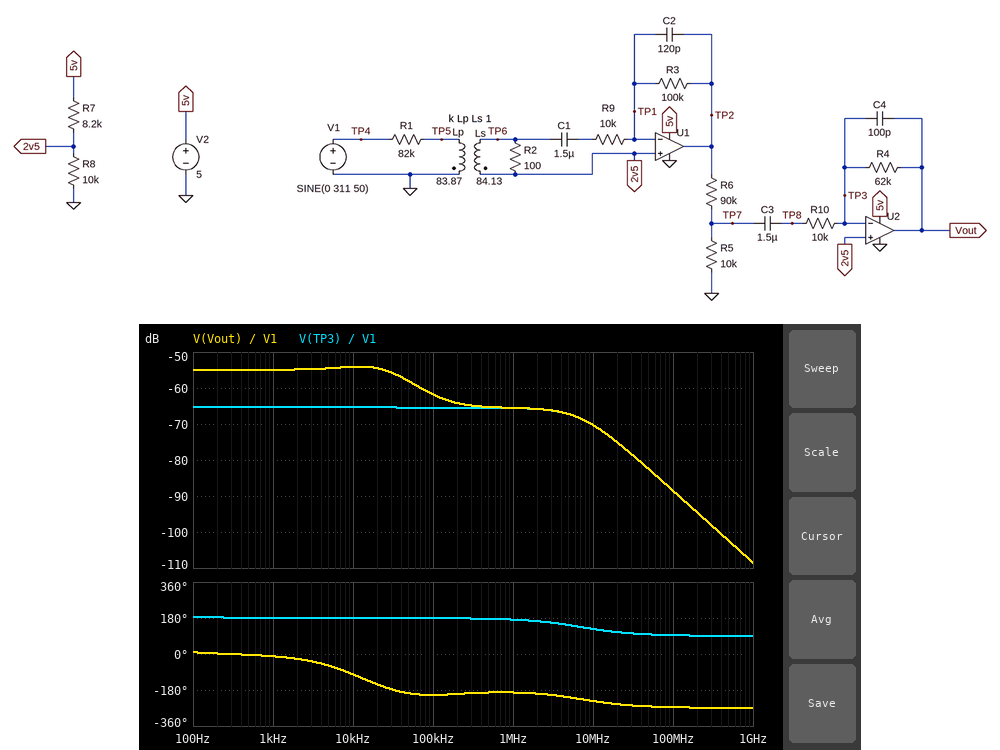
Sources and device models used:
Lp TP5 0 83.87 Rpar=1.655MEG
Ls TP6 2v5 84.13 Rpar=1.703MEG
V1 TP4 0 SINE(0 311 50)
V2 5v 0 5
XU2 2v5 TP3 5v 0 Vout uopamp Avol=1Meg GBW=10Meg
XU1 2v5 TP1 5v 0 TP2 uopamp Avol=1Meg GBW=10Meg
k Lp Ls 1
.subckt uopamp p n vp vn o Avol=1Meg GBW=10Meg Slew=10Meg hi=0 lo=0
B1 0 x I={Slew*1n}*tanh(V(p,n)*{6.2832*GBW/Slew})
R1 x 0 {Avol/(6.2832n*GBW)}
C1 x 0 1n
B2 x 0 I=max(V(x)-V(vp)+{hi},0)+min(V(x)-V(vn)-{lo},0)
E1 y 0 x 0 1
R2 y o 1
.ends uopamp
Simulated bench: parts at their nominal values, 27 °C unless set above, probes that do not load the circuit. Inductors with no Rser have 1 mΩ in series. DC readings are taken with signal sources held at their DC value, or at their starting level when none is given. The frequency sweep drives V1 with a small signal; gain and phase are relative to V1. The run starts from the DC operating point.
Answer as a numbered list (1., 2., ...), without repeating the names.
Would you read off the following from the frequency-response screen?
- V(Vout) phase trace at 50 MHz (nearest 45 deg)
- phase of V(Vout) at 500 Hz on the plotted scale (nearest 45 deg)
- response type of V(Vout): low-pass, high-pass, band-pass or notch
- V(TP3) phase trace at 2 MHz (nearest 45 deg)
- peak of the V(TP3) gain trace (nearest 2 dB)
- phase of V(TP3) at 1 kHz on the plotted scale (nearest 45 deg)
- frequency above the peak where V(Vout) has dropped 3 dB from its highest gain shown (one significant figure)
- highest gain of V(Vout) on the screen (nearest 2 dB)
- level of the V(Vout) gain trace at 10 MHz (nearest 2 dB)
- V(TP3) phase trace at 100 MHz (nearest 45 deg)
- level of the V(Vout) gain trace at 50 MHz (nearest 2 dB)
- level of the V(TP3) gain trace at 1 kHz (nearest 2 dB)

1. -270 deg
2. 0 deg
3. low-pass
4. 180 deg
5. -66 dB
6. 180 deg
7. 40 kHz
8. -54 dB
9. -70 dB
10. 90 deg
11. -82 dB
12. -66 dB
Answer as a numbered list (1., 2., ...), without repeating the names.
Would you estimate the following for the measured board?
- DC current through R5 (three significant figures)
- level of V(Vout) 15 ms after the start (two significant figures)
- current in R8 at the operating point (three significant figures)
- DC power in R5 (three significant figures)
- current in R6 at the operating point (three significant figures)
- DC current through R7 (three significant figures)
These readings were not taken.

1. 27.5 µA
2. 2.4 V
3. 275 µA
4. 7.55 µW
5. 27.5 µA
6. 275 µA
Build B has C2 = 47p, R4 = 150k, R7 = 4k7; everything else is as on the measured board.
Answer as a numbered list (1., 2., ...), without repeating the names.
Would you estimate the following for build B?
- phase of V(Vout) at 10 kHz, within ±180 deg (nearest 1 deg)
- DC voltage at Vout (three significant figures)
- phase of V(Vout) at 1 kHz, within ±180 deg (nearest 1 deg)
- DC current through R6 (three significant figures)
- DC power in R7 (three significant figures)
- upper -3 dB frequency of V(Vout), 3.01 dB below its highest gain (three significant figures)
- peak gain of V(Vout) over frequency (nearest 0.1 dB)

1. -72 deg
2. 3.40 V
3. -7 deg
4. 34.0 µA
5. 544 µW
6. 10.4 kHz
7. -43.9 dB
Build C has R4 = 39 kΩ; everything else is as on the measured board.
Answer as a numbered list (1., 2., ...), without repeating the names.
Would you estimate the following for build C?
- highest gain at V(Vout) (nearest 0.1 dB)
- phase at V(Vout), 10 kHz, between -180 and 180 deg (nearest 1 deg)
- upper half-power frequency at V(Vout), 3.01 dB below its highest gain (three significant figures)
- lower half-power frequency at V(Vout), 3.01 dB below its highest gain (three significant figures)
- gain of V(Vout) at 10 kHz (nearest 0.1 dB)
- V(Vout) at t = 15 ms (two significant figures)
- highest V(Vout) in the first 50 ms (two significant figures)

1. -56.9 dB
2. -103 deg
3. 67.5 kHz
4. 3.76 kHz
5. -57.9 dB
6. 2.6 V
7. 3.0 V
